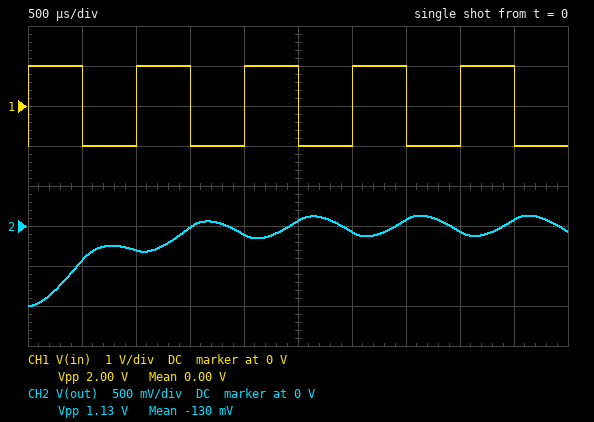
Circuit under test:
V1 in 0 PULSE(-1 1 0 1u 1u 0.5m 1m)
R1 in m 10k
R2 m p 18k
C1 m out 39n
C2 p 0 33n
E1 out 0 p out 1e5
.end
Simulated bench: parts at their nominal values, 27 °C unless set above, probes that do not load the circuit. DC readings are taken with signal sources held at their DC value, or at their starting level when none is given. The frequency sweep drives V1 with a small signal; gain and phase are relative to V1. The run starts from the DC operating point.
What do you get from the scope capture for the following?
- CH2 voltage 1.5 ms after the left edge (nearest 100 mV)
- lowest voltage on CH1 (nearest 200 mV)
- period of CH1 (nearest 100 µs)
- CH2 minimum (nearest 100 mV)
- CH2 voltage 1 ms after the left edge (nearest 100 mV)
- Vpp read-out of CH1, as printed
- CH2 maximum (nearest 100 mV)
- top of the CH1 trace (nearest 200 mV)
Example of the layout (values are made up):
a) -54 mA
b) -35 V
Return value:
a) 0 V
b) -1.0 V
c) 1.0 ms
d) -1.0 V
e) -300 mV
f) 2.00 V
g) 100 mV
h) 1.0 V
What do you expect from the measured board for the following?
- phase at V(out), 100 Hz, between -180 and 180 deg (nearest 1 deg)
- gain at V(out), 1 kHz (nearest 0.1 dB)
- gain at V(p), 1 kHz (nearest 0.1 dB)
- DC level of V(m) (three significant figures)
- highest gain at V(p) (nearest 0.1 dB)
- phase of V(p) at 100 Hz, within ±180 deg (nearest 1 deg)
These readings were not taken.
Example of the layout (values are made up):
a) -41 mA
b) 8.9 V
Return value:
a) -33 deg
b) -20.0 dB
c) -20.0 dB
d) -1.00 V
e) 0 dB
f) -33 deg
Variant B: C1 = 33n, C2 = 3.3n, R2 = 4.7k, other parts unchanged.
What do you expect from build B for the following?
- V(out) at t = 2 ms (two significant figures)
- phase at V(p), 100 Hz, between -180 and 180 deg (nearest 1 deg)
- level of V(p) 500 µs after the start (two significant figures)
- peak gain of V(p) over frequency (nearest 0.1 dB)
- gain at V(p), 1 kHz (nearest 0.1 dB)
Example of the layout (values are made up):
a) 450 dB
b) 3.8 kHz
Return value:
a) -820 mV
b) -2 deg
c) 800 mV
d) 3.9 dB
e) 1.4 dB
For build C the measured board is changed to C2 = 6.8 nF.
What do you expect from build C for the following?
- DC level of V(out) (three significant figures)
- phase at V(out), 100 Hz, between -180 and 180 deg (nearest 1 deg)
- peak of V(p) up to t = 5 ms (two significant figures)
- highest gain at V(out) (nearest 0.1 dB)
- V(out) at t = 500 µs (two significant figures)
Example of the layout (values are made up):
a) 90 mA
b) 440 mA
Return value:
a) -1.00 V
b) -7 deg
c) 1.1 V
d) 2.1 dB
e) 1.0 V
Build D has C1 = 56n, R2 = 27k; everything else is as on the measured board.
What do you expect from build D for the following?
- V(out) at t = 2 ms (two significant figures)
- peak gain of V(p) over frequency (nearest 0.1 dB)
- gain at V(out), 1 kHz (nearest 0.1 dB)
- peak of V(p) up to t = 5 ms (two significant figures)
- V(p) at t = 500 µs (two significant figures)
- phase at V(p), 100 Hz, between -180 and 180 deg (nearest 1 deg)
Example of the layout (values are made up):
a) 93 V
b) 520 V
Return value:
a) -120 mV
b) 0 dB
c) -26.1 dB
d) 68 mV
e) -670 mV
f) -44 deg
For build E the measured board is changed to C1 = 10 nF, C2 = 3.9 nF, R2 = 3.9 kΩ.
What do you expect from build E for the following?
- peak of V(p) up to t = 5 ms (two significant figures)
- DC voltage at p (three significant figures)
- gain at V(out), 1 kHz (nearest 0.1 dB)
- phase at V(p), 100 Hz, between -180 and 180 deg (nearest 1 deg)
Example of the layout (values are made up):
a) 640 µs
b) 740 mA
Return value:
a) 1.1 V
b) -1.00 V
c) 0 dB
d) -2 deg
